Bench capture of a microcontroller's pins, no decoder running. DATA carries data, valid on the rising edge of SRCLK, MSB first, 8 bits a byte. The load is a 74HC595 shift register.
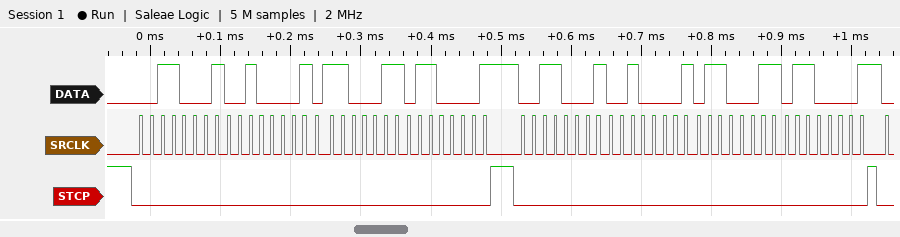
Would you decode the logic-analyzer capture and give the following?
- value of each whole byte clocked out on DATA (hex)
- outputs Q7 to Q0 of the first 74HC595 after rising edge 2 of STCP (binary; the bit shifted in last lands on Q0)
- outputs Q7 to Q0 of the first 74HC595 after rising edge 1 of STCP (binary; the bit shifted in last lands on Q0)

31 21 63 61 31 21 63 61
01100001
01100001
